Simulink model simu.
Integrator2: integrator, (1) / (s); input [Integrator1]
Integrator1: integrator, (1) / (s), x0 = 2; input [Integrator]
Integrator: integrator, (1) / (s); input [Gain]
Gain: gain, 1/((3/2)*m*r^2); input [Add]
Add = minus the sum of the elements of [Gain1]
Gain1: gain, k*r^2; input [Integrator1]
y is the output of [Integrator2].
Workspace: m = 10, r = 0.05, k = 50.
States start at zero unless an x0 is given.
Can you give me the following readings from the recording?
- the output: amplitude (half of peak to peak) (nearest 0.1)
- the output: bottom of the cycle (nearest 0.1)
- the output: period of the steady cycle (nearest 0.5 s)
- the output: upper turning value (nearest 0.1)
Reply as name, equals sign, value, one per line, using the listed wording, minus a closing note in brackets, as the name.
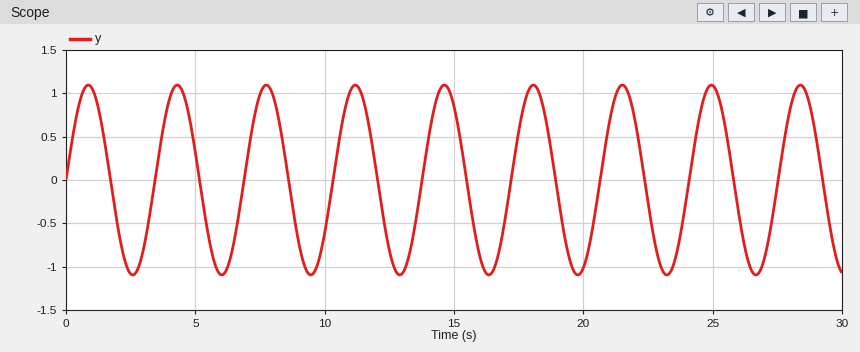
the output: amplitude (half of peak to peak) = 1.1
the output: bottom of the cycle = -1.1
the output: period of the steady cycle = 3.5 s
the output: upper turning value = 1.1
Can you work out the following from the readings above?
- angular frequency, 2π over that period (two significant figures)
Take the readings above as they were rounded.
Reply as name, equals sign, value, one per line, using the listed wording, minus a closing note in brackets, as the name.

angular frequency, 2π over that period = 1.8 rad/s
